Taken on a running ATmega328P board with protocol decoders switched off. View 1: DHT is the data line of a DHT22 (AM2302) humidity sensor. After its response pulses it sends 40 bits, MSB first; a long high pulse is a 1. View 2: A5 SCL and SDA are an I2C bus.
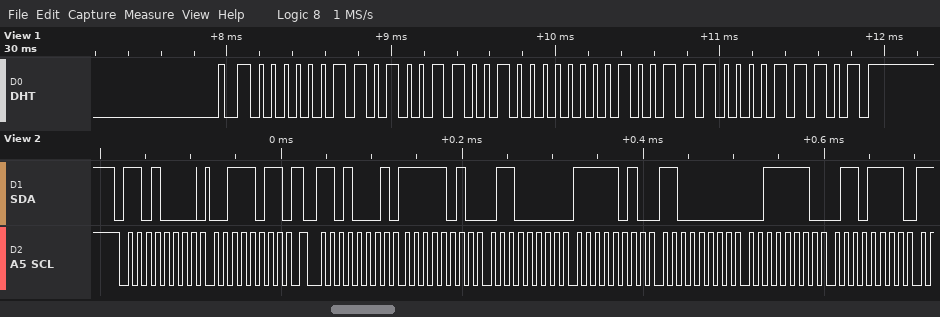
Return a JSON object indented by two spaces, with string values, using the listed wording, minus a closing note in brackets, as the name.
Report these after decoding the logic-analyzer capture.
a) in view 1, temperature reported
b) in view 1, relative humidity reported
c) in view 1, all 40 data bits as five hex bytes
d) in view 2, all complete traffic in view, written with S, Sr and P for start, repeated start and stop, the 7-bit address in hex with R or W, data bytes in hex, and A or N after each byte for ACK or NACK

{
  "in view 1, temperature reported": "-7.8 °C",
  "in view 1, relative humidity reported": "84.4 %",
  "in view 1, all 40 data bits as five hex bytes": "03 4C 80 4E 1D",
  "in view 2, all complete traffic in view, written with S, Sr and P for start, repeated start and stop, the 7-bit address in hex with R or W, data bytes in hex, and A or N after each byte for ACK or NACK": "S 68W A 3B A Sr 68R A FA A 60 A FA A C0 A 3E A 6F A"
}
